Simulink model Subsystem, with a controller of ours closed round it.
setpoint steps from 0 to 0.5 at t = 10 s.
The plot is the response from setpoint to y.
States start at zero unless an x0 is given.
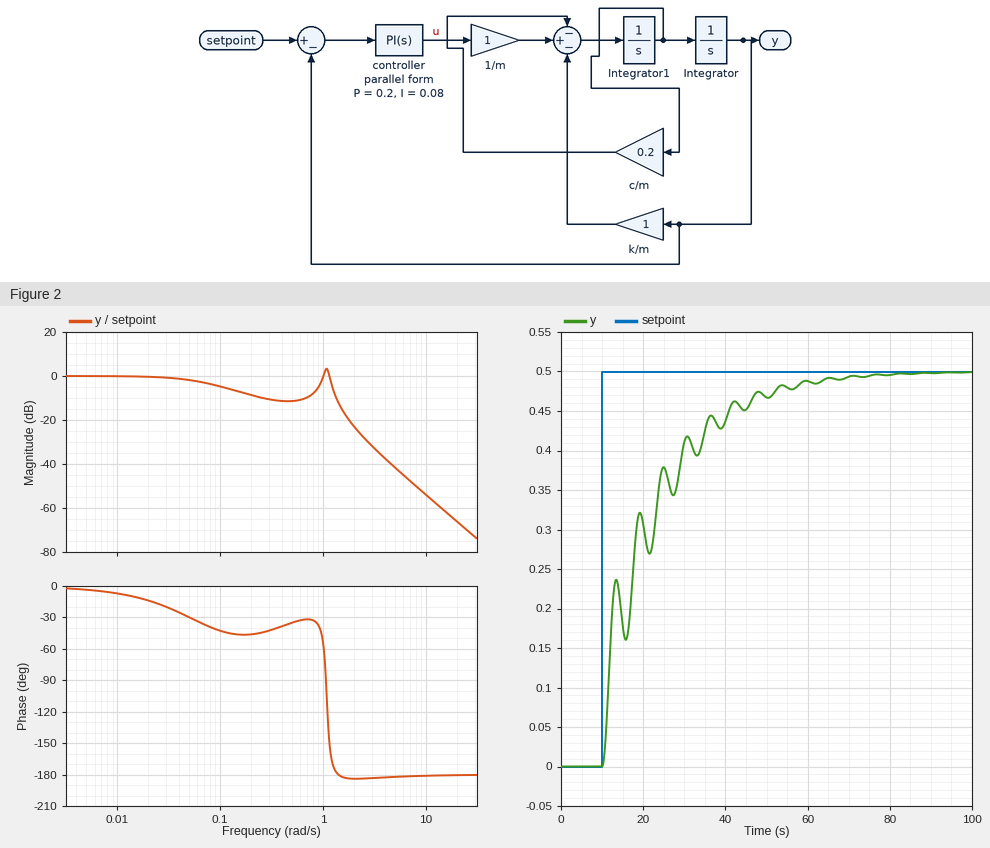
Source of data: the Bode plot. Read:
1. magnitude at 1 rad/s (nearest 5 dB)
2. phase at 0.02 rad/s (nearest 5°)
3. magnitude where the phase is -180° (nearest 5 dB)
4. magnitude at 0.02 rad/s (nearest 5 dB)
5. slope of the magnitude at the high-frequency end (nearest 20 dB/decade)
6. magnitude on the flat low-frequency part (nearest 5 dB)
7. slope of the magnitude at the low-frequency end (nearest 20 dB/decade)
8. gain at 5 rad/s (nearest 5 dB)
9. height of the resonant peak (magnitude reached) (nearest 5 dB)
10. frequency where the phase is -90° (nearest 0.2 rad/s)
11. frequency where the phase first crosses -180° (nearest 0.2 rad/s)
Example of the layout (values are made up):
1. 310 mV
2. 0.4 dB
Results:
1. 0 dB
2. -15°
3. -10 dB
4. 0 dB
5. -40 dB/decade
6. 0 dB
7. 0 dB/decade
8. -40 dB
9. 5 dB
10. 1.0 rad/s
11. 1.4 rad/s
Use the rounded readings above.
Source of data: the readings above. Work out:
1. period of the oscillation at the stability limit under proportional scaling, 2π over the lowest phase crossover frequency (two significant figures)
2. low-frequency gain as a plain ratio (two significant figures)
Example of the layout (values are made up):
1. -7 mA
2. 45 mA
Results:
1. 4.5 s
2. 1.0
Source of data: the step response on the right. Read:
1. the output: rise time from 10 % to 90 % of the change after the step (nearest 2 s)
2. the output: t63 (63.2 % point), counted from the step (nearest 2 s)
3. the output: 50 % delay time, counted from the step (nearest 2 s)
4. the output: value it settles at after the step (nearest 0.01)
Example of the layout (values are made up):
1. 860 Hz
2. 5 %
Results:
1. 30 s
2. 8 s
3. 8 s
4. 0.50
